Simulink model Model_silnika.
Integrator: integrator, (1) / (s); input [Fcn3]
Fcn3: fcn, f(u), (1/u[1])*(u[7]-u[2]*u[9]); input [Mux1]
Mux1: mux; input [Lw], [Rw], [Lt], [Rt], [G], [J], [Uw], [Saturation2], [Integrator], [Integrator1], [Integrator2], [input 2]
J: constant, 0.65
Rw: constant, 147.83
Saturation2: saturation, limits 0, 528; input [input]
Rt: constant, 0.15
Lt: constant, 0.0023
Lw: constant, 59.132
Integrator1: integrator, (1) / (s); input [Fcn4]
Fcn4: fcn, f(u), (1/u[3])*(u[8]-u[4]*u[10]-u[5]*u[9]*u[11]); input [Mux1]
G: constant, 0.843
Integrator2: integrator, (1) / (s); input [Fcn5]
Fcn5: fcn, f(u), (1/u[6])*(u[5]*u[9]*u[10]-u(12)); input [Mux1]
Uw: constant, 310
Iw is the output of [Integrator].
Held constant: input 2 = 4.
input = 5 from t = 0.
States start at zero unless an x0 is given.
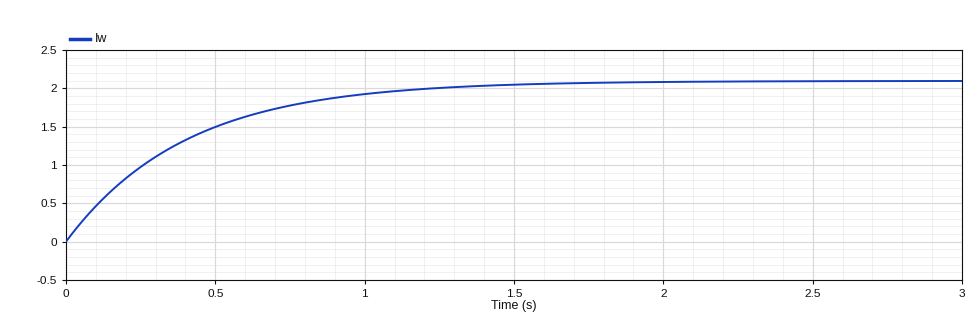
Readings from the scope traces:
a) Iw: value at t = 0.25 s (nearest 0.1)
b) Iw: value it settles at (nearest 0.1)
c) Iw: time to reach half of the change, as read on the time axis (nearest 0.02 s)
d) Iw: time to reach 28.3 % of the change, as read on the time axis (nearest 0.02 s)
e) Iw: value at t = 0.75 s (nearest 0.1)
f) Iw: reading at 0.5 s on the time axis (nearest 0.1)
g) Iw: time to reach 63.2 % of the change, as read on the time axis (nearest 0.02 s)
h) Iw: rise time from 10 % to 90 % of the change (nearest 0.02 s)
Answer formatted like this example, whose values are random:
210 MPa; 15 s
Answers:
1.0; 2.1; 0.28 s; 0.14 s; 1.8; 1.5; 0.40 s; 0.88 s
